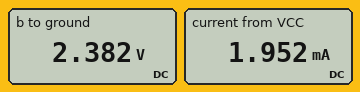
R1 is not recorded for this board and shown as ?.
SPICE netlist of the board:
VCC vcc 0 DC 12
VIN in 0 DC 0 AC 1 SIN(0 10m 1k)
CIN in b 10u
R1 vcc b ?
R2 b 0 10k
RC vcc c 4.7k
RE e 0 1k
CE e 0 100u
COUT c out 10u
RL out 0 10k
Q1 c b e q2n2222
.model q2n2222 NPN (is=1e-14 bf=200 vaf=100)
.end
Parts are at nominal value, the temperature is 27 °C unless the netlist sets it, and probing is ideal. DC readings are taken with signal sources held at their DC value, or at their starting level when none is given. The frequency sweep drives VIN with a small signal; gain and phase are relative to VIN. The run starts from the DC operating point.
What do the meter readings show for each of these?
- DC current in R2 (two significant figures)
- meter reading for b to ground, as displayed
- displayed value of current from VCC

240 µA
2.382 V
1.952 mA
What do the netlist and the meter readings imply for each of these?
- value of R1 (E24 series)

39 kΩ
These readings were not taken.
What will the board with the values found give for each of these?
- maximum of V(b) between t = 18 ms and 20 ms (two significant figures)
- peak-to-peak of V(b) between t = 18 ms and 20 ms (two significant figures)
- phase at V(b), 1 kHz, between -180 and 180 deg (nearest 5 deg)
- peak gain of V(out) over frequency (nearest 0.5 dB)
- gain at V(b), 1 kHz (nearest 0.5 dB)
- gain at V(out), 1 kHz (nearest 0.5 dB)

2.4 V
20 mV
0 deg
46.0 dB
0 dB
46.0 dB
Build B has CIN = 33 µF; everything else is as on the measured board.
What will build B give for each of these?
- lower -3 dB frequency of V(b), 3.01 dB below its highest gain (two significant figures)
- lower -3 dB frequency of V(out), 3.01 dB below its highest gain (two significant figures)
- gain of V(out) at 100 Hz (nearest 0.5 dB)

640 mHz
100 Hz
43.0 dB
